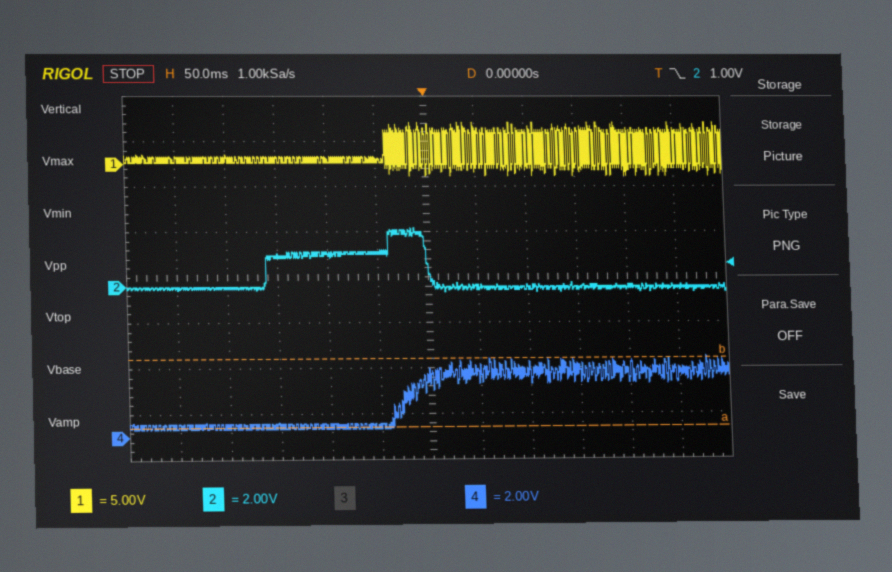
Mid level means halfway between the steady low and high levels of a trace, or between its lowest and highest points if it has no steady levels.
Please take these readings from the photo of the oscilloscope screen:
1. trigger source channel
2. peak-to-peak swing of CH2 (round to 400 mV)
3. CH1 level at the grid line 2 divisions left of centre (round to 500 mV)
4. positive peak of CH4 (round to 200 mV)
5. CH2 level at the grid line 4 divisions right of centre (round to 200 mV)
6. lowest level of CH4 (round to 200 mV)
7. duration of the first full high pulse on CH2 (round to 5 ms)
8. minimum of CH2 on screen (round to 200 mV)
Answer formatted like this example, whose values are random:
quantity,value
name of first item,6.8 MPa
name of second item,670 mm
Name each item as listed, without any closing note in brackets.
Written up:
quantity,value
trigger source channel,CH2
peak-to-peak swing of CH2,2.8 V
CH1 level at the grid line 2 divisions left of centre,500 mV
positive peak of CH4,3.4 V
CH2 level at the grid line 4 divisions right of centre,0.0 V
lowest level of CH4,400 mV
duration of the first full high pulse on CH2,160 ms
minimum of CH2 on screen,-200 mV
